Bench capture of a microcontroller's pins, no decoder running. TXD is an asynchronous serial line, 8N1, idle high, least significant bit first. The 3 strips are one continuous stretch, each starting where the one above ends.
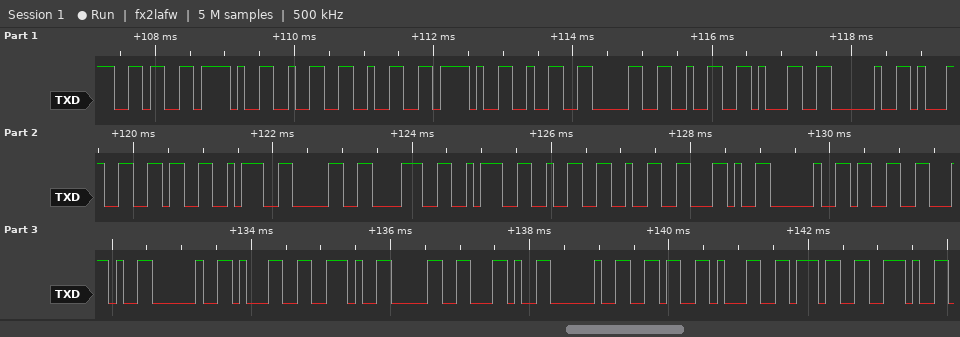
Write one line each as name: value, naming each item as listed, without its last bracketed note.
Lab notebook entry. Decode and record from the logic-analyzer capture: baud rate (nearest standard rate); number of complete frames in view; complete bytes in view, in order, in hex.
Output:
baud rate: 9600 baud
number of complete frames in view: 32
complete bytes in view, in order, in hex: 0x36 0x2F 0x32 0x32 0x2F 0x32 0x30 0x32 0x31 0x20 0x31 0x36 0x3A 0x30 0x38 0x3A 0x32 0x32 0x2C 0x20 0x33 0x2C 0x20 0x31 0x2E 0x30 0x2C 0x20 0x36 0x31 0x37 0x2E
